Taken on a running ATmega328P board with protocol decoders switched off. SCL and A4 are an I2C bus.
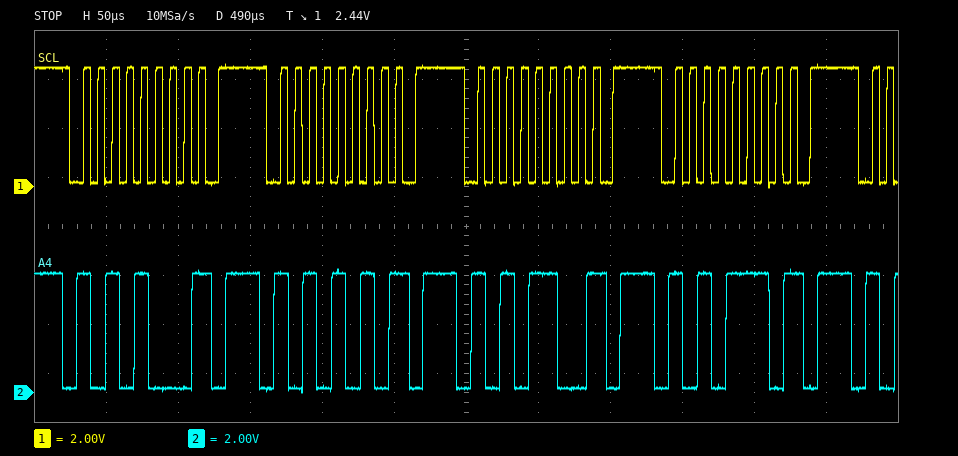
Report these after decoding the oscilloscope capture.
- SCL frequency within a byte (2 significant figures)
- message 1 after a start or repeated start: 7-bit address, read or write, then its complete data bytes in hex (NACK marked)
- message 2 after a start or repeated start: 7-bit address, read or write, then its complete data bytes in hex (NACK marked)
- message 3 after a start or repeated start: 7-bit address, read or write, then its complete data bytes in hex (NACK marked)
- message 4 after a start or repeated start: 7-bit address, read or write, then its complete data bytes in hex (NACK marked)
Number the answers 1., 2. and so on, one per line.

1. 100 kHz
2. 0x54 write NACK
3. 0x55 write NACK
4. 0x56 write NACK
5. 0x57 write NACK
